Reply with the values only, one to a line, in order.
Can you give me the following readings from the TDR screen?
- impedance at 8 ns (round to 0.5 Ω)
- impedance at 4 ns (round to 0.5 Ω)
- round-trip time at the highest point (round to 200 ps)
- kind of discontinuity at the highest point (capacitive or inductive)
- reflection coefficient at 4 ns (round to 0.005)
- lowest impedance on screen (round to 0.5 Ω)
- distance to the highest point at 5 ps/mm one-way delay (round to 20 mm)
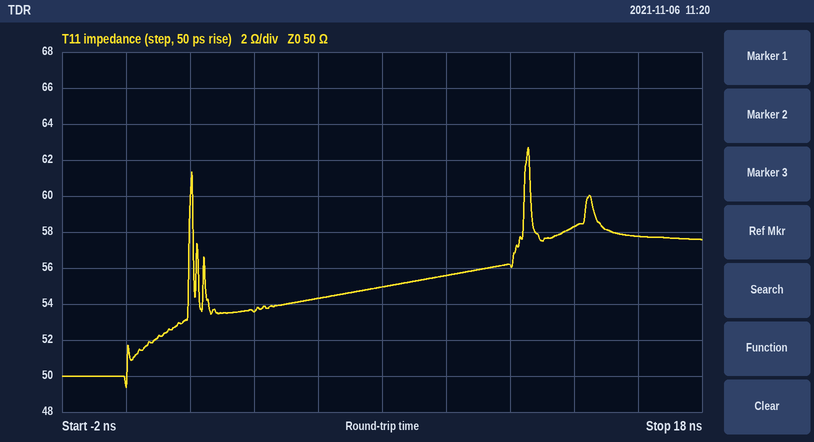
55.0 Ω
53.5 Ω
12.6 ns
inductive
+0.035
49.5 Ω
1.26 m
